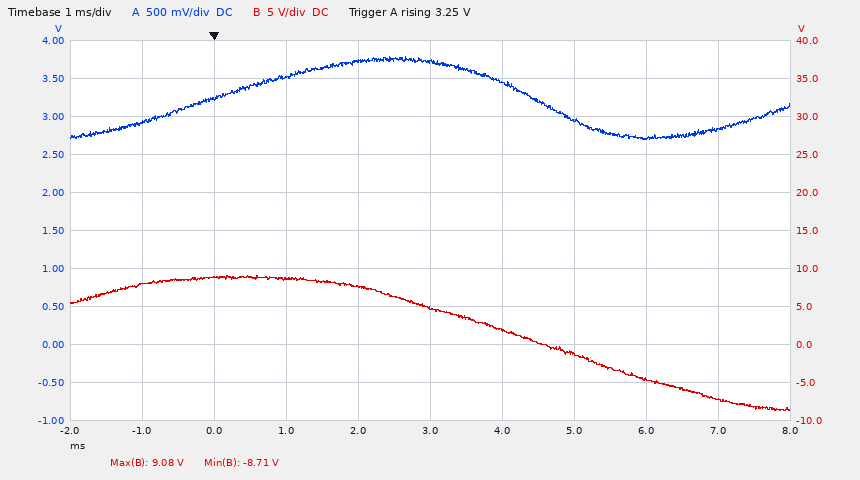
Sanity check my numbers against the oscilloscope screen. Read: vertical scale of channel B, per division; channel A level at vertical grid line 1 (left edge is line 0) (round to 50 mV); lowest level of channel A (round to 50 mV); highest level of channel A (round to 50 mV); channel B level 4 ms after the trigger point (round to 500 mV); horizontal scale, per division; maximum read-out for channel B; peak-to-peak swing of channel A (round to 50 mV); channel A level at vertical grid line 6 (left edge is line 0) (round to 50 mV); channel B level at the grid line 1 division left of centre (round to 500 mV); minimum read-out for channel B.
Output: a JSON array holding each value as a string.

["5 V", "2.90 V", "2.70 V", "3.80 V", "2.0 V", "1 ms", "9.08 V", "1.10 V", "3.45 V", "7.5 V", "-8.71 V"]
